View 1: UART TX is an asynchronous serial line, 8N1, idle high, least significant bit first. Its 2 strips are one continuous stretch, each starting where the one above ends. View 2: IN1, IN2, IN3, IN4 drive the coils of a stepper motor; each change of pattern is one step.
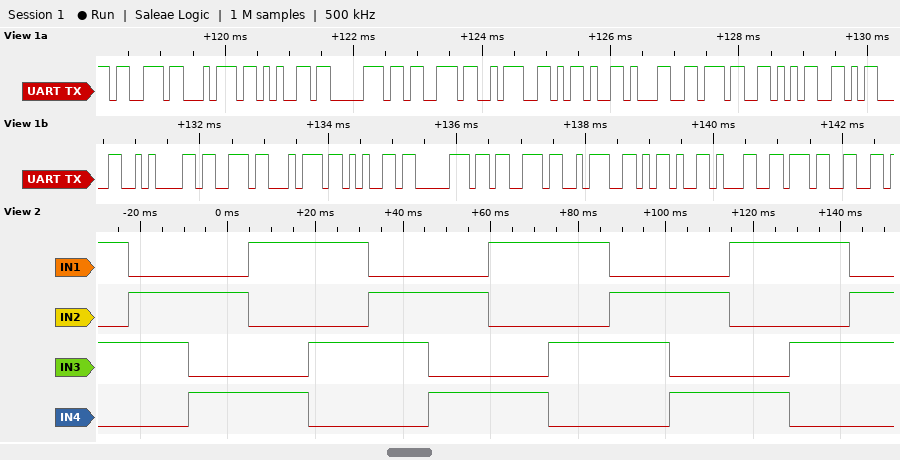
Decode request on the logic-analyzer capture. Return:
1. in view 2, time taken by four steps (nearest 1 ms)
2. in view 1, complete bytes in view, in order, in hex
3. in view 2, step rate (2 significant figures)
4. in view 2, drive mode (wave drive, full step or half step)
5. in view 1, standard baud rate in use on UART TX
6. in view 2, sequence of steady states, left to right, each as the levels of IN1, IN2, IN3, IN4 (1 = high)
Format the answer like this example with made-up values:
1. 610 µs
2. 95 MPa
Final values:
1. 55 ms
2. 0x73 0x74 0x65 0x70 0x73 0x3A 0x2D 0x31 0x37 0x35 0x0D 0x0A 0x73 0x74 0x65 0x70 0x73 0x3A 0x2D 0x31 0x37
3. 73 steps/s
4. full step
5. 9600 baud
6. 1010 0110 0101 1001 1010 0110 0101 1001 1010 0110 0101 1001 1010 0110
